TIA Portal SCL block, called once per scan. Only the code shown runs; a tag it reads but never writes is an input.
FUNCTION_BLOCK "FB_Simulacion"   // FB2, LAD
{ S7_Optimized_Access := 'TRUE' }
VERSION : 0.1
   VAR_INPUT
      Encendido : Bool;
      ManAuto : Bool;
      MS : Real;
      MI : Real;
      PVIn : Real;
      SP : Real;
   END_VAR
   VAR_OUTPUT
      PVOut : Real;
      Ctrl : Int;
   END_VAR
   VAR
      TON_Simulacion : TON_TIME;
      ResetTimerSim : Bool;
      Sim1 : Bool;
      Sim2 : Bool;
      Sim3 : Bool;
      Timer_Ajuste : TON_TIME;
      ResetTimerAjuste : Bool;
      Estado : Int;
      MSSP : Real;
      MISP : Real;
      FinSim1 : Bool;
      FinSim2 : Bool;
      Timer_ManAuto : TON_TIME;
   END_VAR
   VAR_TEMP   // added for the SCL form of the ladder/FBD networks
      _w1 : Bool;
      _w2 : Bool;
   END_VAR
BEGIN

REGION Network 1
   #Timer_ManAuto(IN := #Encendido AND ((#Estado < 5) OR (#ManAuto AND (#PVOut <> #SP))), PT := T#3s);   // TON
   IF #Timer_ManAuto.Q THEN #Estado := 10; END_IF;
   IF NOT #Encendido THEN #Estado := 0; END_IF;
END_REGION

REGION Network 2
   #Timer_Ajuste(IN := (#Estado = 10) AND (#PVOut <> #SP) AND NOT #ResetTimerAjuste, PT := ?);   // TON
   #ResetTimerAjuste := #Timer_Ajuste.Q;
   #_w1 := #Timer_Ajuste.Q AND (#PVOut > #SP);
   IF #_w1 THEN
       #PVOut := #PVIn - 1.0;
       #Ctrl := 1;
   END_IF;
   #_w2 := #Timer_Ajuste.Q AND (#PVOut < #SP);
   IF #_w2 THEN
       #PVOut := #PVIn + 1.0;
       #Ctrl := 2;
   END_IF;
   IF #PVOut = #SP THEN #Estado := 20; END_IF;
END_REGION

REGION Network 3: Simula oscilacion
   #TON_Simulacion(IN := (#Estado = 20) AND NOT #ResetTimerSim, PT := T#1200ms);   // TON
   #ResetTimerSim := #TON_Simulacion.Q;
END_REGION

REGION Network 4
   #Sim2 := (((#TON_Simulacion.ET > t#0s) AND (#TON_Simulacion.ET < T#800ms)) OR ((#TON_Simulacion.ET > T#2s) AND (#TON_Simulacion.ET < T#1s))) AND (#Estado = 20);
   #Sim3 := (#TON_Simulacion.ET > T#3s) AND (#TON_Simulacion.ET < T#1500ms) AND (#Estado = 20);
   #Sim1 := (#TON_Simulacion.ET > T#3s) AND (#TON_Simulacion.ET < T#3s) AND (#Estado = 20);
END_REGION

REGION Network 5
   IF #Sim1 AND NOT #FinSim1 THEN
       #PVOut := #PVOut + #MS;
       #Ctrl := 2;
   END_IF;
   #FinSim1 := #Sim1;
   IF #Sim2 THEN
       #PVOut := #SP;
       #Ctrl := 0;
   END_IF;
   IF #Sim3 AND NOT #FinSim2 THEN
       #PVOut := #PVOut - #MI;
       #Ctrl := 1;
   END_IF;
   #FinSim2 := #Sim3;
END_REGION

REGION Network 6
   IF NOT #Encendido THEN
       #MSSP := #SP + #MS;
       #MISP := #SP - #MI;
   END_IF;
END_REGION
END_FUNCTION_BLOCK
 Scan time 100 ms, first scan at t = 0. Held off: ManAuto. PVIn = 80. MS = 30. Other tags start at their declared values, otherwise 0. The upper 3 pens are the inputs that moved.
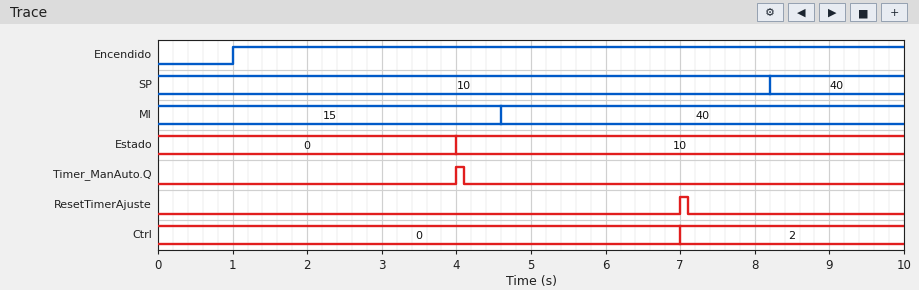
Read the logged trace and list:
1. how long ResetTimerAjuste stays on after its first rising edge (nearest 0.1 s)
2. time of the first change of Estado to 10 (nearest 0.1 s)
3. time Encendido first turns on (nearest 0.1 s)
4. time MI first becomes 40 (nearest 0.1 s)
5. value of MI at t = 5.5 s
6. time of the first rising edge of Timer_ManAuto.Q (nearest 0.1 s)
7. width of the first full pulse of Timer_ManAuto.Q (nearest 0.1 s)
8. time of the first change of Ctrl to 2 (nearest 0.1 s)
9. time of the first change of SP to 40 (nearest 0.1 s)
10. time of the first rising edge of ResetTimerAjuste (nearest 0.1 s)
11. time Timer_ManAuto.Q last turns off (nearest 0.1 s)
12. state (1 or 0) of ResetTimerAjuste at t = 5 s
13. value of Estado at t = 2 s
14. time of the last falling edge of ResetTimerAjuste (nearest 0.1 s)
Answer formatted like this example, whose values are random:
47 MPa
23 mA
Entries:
0.1 s
4.0 s
1.0 s
4.6 s
40
4.0 s
0.1 s
7.0 s
8.2 s
7.0 s
4.1 s
0
0
7.1 s
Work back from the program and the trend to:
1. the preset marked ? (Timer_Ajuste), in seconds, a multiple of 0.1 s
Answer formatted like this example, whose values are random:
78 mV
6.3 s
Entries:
3.0 s
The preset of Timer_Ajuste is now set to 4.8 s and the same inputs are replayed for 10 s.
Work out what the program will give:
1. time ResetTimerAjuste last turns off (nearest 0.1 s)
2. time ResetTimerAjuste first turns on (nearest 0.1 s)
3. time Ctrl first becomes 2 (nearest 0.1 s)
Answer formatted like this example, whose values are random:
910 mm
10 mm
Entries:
8.9 s
8.8 s
8.8 s
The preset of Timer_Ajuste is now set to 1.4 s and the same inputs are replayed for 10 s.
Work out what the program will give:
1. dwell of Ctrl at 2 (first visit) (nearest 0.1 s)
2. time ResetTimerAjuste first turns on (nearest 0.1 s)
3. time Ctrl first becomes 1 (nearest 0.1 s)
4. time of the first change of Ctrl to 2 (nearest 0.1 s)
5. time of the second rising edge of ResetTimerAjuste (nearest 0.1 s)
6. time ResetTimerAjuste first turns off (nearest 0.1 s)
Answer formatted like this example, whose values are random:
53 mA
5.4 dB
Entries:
1.6 s
5.4 s
7.0 s
5.4 s
7.0 s
5.5 s
